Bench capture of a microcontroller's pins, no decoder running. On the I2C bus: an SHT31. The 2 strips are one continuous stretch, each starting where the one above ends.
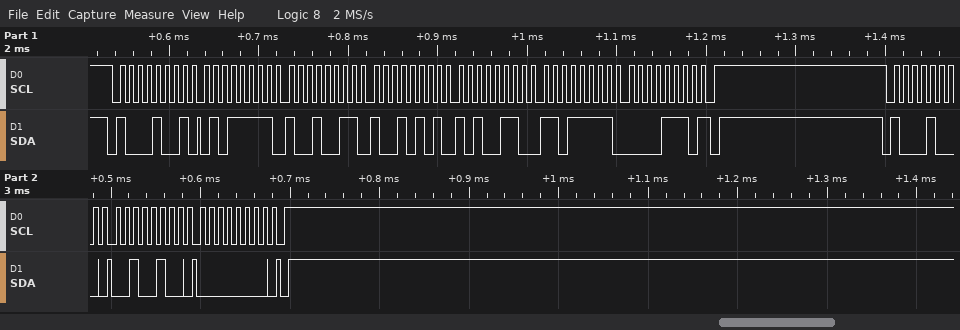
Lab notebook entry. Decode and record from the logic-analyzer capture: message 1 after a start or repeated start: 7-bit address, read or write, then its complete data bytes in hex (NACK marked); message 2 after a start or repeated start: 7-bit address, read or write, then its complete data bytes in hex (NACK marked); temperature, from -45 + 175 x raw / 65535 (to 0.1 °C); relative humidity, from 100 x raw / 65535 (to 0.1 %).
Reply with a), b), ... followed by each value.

a) 0x44 read: 5F 93 95 A6 DF 0E NACK
b) 0x44 write: 24 00
c) 20.3 °C
d) 65.2 %
